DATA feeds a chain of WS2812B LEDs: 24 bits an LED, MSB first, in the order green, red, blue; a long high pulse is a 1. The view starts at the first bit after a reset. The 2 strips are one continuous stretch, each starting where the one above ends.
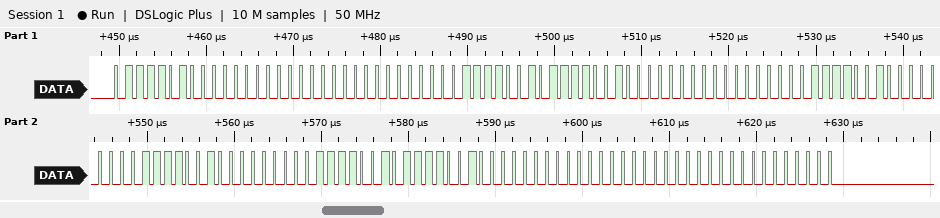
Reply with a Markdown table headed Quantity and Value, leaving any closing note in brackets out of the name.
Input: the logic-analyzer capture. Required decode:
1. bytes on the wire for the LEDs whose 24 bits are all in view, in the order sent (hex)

| Quantity | Value |
|---|---|
| bytes on the wire for the LEDs whose 24 bits are all in view, in the order sent | 7A 00 00 00 F2 F2 00 00 F2 00 F2 00 F2 F2 00 00 00 00 |
